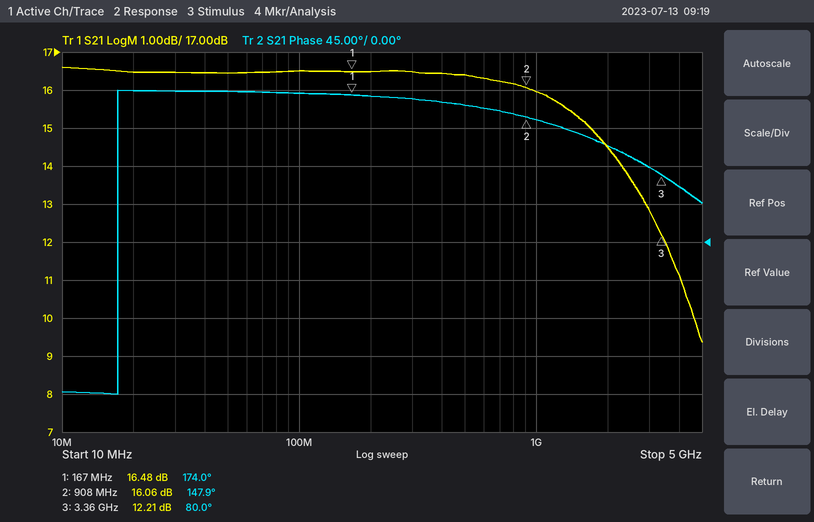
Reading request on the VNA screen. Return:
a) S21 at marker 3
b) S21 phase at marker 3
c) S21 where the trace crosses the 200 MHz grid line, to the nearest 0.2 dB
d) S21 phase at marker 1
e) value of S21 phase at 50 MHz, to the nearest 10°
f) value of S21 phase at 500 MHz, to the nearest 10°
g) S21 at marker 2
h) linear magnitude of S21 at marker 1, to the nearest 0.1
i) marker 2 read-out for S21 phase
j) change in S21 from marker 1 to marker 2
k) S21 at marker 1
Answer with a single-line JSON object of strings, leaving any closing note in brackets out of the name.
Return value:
{"S21 at marker 3": "12.21 dB", "S21 phase at marker 3": "80.0°", "S21 where the trace crosses the 200 MHz grid line, to the nearest 0.2 dB": "16.4 dB", "S21 phase at marker 1": "174.0°", "value of S21 phase at 50 MHz, to the nearest 10°": "180°", "value of S21 phase at 500 MHz, to the nearest 10°": "160°", "S21 at marker 2": "16.06 dB", "linear magnitude of S21 at marker 1, to the nearest 0.1": "6.7", "marker 2 read-out for S21 phase": "147.9°", "change in S21 from marker 1 to marker 2": "-0.42 dB", "S21 at marker 1": "16.48 dB"}
